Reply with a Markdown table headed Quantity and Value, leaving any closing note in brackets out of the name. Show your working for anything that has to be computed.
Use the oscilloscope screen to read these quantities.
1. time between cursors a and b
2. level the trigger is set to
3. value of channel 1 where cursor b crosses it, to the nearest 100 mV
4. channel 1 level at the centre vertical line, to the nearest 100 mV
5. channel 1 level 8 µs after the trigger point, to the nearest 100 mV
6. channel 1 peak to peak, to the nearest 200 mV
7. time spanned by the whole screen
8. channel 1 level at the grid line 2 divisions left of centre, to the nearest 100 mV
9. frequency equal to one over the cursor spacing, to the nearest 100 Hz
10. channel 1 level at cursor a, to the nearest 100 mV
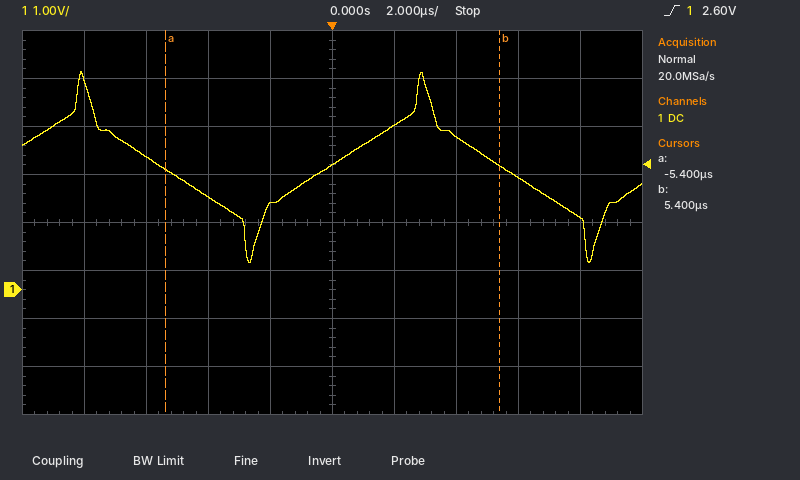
| Quantity | Value |
|---|---|
| time between cursors a and b | 5.4 µs − (-5.4 µs) = 10.8 µs |
| level the trigger is set to | 2.60 V |
| value of channel 1 where cursor b crosses it, to the nearest 100 mV | 2.6 V |
| channel 1 level at the centre vertical line, to the nearest 100 mV | 2.6 V |
| channel 1 level 8 µs after the trigger point, to the nearest 100 mV | 1.5 V |
| channel 1 peak to peak, to the nearest 200 mV | 4.0 V |
| time spanned by the whole screen | 20 µs |
| channel 1 level at the grid line 2 divisions left of centre, to the nearest 100 mV | 1.9 V |
| frequency equal to one over the cursor spacing, to the nearest 100 Hz | 1 / 10.8 µs ≈ 92.6 kHz |
| channel 1 level at cursor a, to the nearest 100 mV | 2.5 V |
